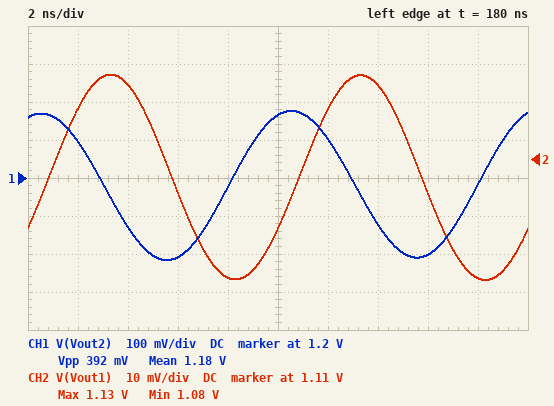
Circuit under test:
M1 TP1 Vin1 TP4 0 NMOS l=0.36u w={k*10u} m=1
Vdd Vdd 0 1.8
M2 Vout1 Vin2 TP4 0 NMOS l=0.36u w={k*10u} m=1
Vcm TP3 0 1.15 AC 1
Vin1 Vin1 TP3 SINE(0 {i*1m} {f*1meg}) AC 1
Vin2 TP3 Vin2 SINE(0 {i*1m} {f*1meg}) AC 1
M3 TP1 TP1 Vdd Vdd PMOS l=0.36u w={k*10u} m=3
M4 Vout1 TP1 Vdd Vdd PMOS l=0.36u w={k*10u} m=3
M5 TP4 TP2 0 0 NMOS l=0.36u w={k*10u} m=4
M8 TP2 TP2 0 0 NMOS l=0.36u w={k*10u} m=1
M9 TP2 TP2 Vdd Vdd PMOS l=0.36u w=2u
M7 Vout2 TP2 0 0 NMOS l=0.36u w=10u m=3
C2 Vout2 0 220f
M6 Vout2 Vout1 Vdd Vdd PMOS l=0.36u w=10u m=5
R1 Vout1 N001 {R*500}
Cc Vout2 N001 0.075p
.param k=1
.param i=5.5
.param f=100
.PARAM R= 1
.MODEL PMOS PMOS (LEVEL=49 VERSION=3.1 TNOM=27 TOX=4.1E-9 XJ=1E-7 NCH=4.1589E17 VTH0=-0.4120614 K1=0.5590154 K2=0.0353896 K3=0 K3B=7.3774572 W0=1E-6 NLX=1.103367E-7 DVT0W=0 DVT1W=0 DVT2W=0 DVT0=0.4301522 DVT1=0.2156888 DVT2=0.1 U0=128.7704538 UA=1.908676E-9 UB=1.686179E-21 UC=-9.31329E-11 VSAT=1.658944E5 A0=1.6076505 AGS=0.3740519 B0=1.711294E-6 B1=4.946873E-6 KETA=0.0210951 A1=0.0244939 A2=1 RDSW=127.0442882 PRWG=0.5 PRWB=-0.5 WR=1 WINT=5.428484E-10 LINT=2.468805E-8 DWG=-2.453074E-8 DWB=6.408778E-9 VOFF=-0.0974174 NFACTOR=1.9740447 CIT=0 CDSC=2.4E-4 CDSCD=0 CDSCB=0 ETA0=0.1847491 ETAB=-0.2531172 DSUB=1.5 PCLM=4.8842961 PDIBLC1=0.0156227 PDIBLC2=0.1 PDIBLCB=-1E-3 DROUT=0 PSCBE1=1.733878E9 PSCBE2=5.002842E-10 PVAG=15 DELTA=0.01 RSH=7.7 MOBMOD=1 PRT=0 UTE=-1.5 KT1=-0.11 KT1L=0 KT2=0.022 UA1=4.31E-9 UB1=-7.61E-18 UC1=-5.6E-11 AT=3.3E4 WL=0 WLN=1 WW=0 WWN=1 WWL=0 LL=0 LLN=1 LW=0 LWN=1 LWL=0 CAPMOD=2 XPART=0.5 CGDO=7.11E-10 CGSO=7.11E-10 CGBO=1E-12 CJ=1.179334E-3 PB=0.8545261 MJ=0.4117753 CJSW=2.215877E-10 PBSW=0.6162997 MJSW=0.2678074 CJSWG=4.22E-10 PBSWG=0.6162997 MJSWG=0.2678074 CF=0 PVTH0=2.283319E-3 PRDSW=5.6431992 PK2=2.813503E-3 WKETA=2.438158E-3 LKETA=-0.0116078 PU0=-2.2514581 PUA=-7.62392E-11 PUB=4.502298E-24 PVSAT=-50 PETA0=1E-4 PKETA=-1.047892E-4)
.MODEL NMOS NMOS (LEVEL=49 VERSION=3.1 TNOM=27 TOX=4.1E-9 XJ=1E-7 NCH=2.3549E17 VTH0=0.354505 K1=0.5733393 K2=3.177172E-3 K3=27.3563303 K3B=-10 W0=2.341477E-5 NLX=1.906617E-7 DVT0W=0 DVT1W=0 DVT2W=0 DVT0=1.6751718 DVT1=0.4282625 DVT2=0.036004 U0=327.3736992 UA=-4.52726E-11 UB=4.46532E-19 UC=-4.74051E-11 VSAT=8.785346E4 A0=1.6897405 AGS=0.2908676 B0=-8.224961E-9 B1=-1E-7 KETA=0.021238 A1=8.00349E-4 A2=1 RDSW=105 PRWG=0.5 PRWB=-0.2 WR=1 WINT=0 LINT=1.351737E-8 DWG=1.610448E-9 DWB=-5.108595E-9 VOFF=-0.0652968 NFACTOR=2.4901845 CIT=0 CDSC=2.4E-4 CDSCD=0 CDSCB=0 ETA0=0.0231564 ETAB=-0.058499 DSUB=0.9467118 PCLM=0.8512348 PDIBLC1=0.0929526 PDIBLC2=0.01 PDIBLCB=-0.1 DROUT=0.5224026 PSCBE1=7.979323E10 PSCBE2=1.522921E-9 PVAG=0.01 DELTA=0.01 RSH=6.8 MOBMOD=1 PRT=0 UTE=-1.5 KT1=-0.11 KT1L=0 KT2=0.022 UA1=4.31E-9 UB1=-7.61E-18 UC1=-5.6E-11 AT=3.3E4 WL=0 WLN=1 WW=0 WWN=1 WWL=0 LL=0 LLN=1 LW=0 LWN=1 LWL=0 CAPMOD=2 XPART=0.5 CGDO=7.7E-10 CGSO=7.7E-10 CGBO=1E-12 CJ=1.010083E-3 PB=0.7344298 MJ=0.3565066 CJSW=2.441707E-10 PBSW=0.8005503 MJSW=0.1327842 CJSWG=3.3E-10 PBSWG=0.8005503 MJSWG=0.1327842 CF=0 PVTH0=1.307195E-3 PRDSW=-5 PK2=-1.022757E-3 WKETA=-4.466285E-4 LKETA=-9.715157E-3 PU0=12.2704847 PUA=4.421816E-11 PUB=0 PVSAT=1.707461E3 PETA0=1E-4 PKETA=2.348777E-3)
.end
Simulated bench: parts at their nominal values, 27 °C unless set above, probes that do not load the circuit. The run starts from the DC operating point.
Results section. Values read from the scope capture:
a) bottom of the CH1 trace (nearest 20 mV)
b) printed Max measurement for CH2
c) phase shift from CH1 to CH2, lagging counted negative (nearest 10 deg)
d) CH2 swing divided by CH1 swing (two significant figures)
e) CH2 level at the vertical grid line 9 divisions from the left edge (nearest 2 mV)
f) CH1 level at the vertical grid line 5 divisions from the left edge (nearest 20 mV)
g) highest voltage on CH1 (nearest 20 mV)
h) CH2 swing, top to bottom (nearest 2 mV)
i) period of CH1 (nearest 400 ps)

980 mV
1.13 V
-100 deg
0.14
1.078 V
1.36 V
1.38 V
54 mV
10.0 ns
